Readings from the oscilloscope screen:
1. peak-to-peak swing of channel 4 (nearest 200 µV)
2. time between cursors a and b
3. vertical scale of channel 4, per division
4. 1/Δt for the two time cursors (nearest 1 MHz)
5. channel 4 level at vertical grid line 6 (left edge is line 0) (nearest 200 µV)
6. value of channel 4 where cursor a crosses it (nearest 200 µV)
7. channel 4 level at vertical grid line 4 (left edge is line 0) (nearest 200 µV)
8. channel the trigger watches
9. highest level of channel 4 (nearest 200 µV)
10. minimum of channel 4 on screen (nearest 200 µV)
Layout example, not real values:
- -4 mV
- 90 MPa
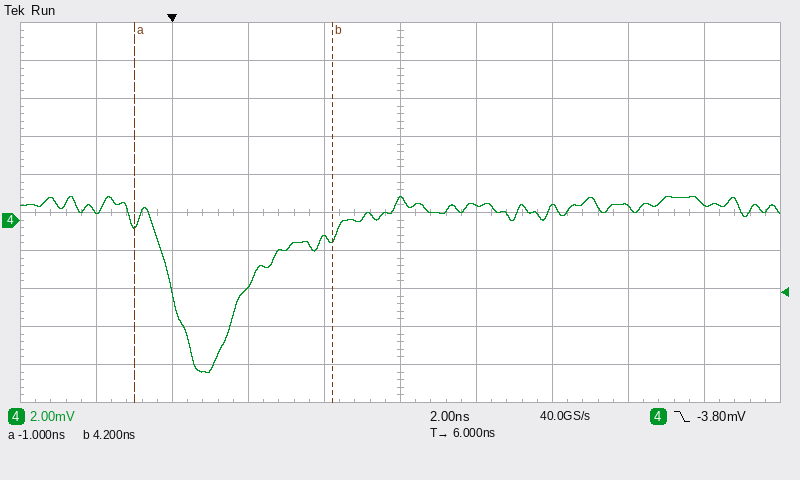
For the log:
- 9.2 mV
- 5.2 ns
- 2 mV
- 192 MHz
- 800 µV
- -200 µV
- -1.0 mV
- channel 4
- 1.2 mV
- -8.0 mV
